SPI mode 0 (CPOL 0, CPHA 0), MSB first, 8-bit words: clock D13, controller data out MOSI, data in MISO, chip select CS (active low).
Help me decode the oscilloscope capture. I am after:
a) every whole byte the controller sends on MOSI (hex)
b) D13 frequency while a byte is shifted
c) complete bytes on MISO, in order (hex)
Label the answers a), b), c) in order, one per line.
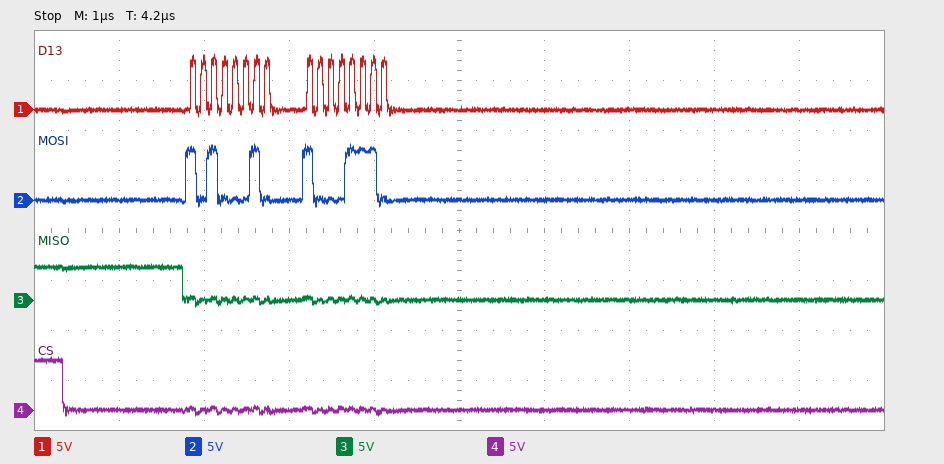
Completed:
a) A2 8E
b) 8 MHz
c) 00 00
